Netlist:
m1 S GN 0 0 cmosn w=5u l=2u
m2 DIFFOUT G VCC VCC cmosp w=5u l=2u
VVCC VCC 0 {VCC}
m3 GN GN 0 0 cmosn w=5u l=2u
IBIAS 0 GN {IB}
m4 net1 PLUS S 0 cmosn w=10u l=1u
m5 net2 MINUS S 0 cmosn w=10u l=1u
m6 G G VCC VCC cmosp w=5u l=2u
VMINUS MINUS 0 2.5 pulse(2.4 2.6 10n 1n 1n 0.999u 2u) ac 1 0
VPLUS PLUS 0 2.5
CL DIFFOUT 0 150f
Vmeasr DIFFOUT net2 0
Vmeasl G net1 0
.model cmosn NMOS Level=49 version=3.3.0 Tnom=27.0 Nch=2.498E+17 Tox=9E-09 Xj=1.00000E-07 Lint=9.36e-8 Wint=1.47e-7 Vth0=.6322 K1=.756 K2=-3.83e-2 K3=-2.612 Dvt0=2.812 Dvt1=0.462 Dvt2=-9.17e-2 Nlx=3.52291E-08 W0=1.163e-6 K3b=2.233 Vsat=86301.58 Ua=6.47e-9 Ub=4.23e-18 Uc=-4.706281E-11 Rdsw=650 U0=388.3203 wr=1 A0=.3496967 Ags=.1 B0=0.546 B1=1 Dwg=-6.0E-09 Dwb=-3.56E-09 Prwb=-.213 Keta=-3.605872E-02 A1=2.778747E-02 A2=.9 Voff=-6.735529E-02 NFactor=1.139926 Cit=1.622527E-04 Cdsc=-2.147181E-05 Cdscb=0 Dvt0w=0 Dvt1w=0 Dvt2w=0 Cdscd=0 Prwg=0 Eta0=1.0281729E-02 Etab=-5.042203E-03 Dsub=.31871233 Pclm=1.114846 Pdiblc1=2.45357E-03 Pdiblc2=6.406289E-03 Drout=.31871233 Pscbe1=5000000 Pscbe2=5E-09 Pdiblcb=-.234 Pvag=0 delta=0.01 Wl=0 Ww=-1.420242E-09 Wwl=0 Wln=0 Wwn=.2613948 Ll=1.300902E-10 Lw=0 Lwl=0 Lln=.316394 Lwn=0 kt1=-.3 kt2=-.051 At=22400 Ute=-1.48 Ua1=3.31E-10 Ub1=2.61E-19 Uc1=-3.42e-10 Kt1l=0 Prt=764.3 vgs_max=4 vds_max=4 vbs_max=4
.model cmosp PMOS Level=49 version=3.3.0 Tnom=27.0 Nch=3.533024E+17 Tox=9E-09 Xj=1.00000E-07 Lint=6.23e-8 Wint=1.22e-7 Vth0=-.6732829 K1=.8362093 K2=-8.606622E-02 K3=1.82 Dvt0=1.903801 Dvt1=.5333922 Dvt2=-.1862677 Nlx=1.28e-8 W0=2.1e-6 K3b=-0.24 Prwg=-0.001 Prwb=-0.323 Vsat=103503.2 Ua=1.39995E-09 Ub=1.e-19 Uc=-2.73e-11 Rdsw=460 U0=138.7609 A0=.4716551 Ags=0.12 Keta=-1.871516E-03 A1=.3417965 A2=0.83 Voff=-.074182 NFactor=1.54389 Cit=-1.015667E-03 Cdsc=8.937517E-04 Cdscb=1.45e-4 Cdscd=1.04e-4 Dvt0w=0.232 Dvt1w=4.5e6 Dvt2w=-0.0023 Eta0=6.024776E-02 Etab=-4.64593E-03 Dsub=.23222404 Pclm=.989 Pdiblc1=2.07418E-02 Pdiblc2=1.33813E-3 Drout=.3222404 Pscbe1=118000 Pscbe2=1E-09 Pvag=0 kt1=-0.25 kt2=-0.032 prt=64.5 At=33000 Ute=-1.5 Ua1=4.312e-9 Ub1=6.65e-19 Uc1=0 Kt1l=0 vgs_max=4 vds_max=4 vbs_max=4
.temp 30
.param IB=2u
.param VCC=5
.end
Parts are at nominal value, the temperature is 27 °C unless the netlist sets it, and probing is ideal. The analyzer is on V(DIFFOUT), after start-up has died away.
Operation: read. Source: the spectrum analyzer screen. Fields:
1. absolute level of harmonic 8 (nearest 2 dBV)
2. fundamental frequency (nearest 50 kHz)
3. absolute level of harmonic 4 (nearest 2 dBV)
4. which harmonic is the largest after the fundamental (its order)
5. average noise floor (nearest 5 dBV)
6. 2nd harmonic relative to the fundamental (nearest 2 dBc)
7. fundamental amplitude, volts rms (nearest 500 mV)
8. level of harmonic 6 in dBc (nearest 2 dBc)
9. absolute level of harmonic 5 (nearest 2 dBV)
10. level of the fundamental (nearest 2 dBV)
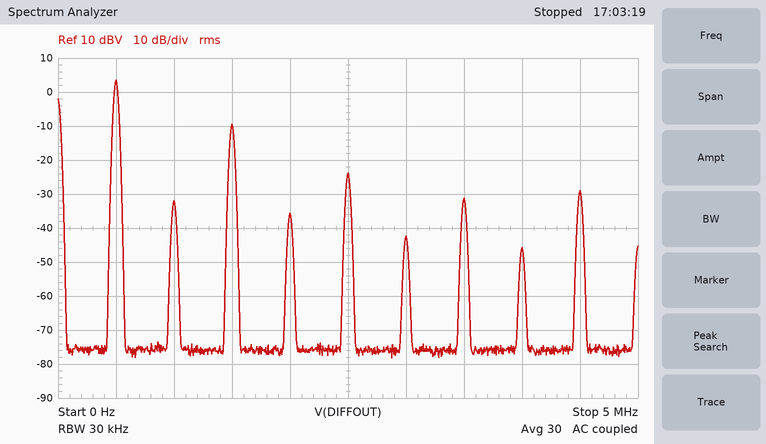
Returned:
-46 dBV
500 kHz
-36 dBV
3
-75 dBV
-36 dBc
1.5 V
-46 dBc
-24 dBV
4 dBV
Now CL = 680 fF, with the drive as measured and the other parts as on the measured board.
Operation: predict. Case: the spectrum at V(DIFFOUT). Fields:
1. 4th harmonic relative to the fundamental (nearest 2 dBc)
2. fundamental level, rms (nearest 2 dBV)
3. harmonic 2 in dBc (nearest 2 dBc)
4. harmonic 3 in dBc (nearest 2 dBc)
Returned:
-46 dBc
-4 dBV
-40 dBc
-20 dBc
